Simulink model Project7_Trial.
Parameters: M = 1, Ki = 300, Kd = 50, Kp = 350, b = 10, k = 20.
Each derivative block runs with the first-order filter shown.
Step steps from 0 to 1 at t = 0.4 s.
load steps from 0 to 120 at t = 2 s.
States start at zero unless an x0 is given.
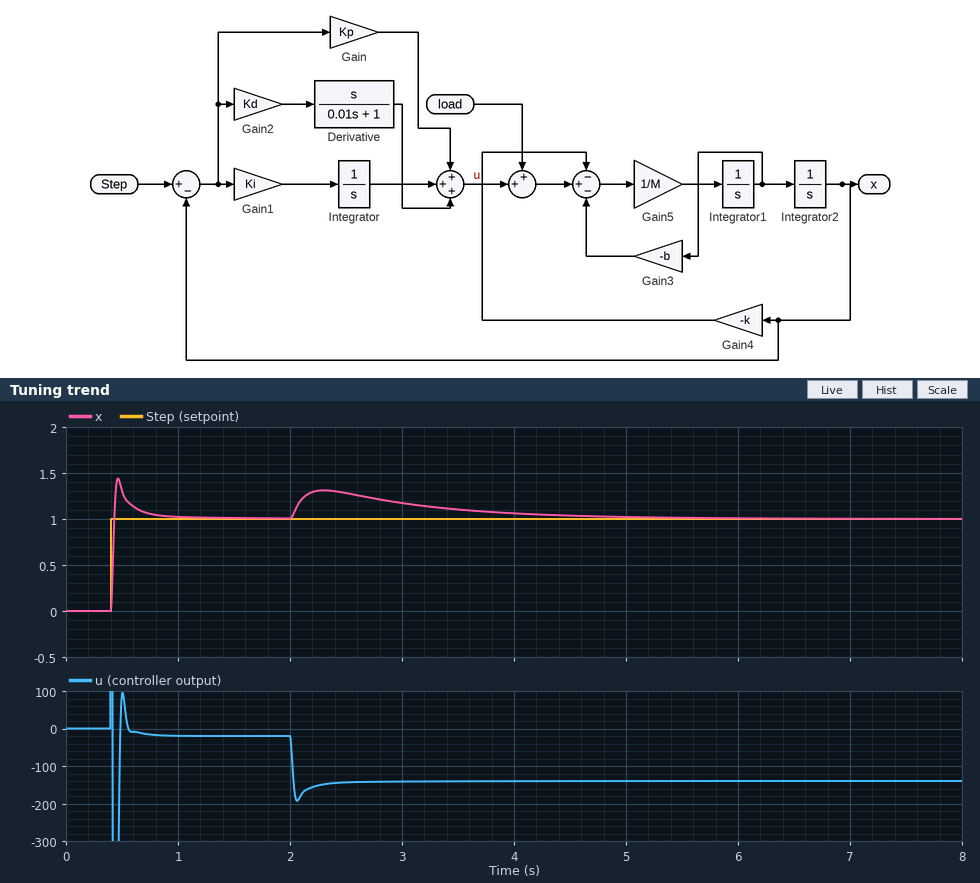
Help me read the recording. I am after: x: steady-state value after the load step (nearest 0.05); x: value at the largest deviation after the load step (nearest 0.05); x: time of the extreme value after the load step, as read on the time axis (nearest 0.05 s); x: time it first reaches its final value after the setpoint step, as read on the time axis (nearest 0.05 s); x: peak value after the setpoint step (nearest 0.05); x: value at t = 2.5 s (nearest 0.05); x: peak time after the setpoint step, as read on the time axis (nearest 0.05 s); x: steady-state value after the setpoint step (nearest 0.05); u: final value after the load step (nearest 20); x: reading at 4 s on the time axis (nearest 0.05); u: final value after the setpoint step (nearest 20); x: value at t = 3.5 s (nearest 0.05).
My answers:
1.00
1.30
2.30 s
0.45 s
1.45
1.30
0.45 s
1.00
-140
1.05
-20
1.10
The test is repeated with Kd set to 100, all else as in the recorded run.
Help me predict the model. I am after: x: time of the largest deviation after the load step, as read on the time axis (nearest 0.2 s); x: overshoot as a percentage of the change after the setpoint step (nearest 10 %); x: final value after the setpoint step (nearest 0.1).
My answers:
2.6 s
40 %
1.0
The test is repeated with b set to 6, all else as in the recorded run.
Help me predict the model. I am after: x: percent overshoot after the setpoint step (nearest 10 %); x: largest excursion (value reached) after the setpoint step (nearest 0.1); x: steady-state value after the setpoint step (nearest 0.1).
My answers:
30 %
1.3
1.0
